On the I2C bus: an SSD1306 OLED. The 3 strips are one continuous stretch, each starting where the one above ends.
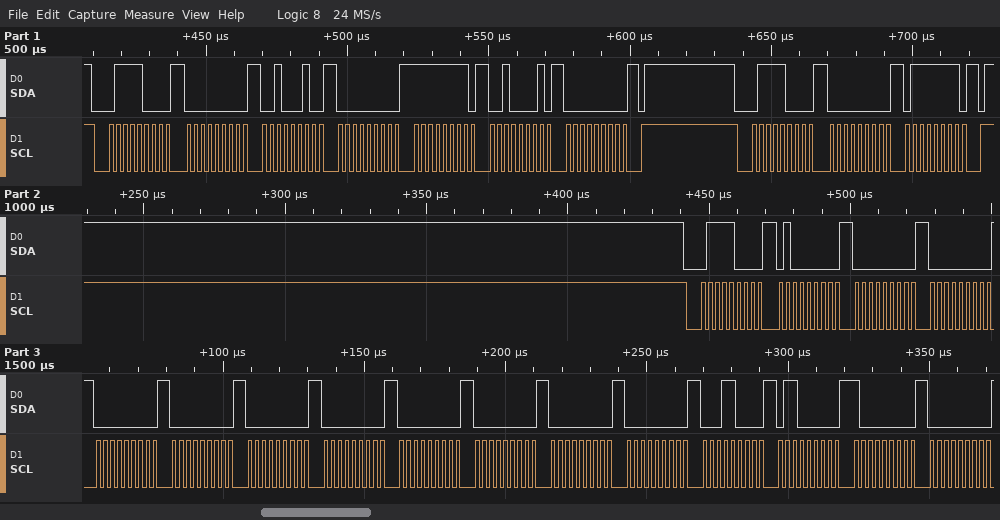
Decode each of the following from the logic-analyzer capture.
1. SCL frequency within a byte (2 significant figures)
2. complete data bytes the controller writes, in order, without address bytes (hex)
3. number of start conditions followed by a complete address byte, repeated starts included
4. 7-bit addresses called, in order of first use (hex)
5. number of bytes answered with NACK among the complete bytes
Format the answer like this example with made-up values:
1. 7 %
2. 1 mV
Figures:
1. 400 kHz
2. 00 22 00 FF 21 00 00 7F 40 00 00 00 00 00 00 00 00 00 00 18 60 80 00
3. 3
4. 0x3C
5. 0
